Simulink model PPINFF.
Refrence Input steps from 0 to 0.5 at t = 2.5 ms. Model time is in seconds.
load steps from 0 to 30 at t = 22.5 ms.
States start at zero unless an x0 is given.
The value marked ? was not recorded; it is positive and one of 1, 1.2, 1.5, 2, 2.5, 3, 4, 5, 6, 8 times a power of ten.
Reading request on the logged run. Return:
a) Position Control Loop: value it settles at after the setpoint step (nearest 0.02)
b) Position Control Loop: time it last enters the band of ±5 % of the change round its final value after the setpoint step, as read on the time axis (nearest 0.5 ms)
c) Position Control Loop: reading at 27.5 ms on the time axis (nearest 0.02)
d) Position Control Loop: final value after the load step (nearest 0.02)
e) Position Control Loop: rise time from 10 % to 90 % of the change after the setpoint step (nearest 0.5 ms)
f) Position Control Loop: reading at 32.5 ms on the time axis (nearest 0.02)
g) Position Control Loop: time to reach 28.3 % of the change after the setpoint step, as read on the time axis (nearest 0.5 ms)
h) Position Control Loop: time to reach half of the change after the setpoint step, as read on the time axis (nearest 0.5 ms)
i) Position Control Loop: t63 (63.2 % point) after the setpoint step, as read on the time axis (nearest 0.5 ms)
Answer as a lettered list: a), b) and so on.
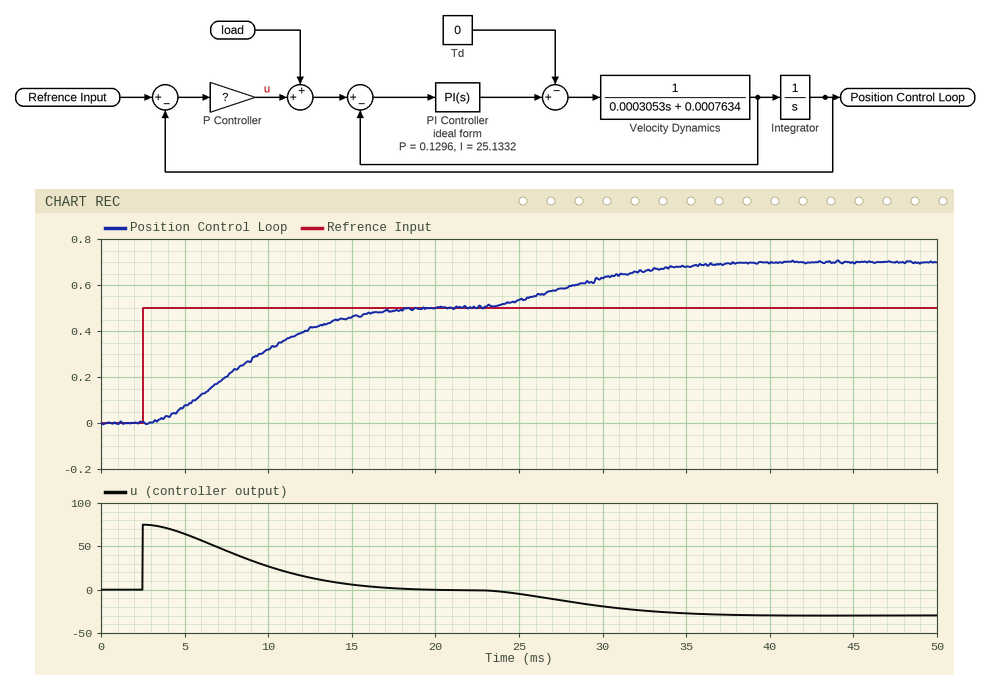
a) 0.50
b) 16.0 ms
c) 0.58
d) 0.70
e) 10.0 ms
f) 0.66
g) 6.5 ms
h) 8.5 ms
i) 10.0 ms
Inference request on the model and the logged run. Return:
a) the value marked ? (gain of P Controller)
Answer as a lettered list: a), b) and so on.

a) 150
